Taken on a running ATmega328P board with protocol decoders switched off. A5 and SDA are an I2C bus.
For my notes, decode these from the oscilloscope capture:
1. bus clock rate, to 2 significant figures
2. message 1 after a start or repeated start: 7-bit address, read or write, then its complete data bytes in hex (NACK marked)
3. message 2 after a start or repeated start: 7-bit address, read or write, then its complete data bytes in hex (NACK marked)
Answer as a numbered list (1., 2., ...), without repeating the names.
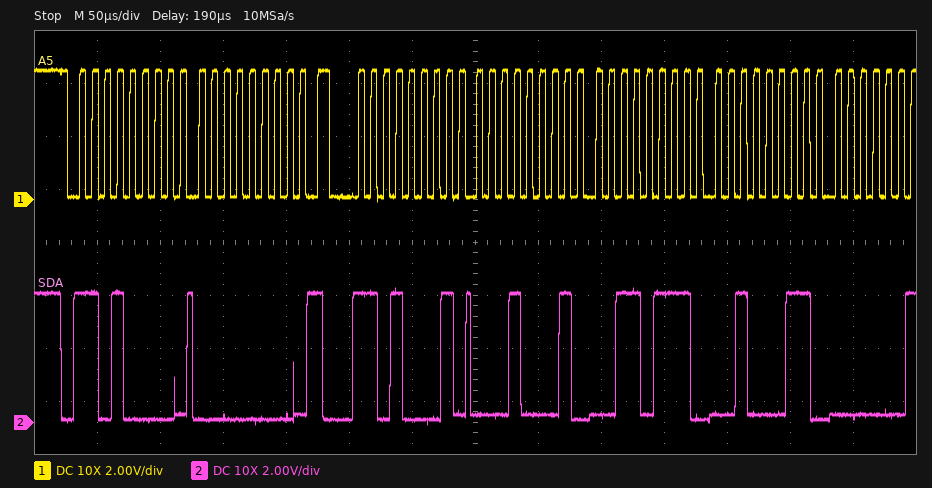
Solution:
1. 100 kHz
2. 0x68 write: 00
3. 0x68 read: 11 37 23
